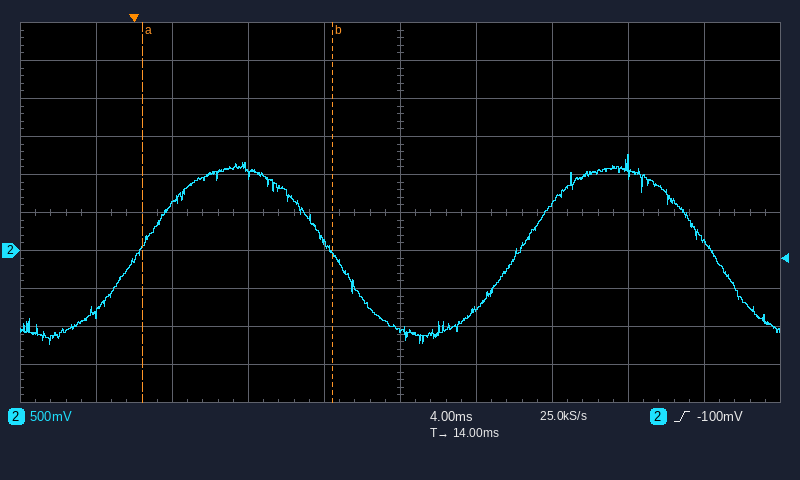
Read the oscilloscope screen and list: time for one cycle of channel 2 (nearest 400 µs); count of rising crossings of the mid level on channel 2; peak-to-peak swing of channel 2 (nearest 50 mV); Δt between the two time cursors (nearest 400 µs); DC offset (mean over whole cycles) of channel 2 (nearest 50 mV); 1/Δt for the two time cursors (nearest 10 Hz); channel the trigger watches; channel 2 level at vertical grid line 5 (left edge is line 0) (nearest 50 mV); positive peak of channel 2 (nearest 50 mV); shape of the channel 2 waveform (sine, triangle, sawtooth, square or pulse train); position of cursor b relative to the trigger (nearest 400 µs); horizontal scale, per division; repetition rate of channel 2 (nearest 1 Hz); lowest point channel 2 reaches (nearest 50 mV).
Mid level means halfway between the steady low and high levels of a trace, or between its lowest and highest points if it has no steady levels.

20.0 ms
2
2.50 V
10.0 ms
0 mV
100 Hz
channel 2
-1.05 V
1.25 V
sine
+10.4 ms
4 ms
50 Hz
-1.25 V
